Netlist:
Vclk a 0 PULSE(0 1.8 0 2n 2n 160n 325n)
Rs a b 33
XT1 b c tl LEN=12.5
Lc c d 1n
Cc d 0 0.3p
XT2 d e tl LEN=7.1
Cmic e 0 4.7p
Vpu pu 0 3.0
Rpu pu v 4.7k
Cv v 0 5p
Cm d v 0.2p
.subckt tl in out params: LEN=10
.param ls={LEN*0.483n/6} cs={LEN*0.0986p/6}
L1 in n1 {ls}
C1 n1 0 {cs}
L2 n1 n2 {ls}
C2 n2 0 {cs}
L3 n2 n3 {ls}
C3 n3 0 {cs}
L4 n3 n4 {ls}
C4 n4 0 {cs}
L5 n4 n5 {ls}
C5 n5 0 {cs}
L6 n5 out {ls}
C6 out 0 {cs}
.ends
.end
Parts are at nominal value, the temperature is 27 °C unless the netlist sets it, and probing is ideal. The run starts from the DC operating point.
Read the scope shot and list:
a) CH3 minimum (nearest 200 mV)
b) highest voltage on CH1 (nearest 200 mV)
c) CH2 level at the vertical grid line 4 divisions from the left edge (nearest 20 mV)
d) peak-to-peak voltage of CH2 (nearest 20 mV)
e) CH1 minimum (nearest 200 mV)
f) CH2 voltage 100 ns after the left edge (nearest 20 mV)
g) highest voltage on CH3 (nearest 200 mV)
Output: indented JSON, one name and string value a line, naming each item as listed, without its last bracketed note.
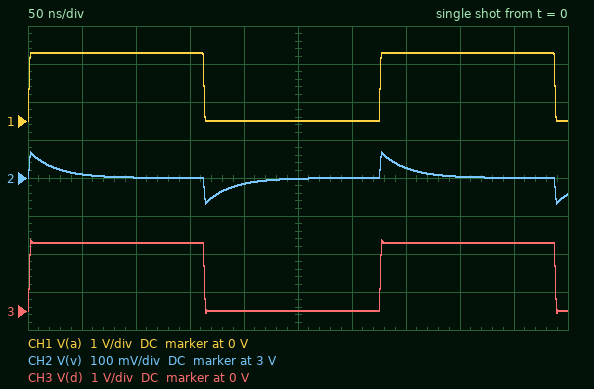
{
  "CH3 minimum": "0 V",
  "highest voltage on CH1": "1.8 V",
  "CH2 level at the vertical grid line 4 divisions from the left edge": "2.98 V",
  "peak-to-peak voltage of CH2": "140 mV",
  "CH1 minimum": "0 V",
  "CH2 voltage 100 ns after the left edge": "3.00 V",
  "highest voltage on CH3": "1.8 V"
}
